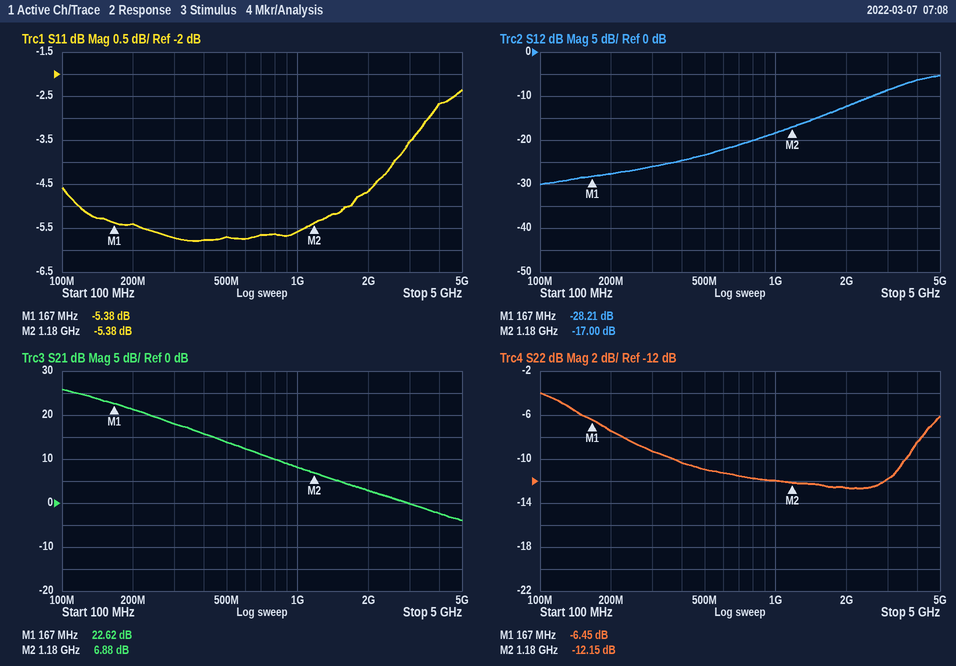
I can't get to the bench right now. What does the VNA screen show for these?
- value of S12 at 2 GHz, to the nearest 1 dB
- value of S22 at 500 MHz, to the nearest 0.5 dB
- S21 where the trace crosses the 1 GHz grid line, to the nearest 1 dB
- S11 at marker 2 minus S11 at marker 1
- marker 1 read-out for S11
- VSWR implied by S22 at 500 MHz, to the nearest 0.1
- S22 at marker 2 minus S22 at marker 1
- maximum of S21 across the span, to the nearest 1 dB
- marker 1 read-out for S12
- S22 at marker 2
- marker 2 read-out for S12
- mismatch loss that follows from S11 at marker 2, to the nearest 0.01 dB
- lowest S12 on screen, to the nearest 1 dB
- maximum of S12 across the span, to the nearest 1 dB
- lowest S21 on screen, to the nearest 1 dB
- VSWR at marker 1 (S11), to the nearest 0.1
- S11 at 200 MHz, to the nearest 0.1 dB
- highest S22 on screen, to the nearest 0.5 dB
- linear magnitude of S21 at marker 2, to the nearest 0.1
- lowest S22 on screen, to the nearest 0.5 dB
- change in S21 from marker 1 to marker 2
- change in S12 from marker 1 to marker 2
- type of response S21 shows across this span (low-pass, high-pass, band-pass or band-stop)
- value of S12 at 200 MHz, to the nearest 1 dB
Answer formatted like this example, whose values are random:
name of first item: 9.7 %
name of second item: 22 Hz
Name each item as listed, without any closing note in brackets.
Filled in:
value of S12 at 2 GHz, to the nearest 1 dB: -12 dB
value of S22 at 500 MHz, to the nearest 0.5 dB: -11.0 dB
S21 where the trace crosses the 1 GHz grid line, to the nearest 1 dB: 8 dB
S11 at marker 2 minus S11 at marker 1: 0.00 dB
marker 1 read-out for S11: -5.38 dB
VSWR implied by S22 at 500 MHz, to the nearest 0.1: 1.8
S22 at marker 2 minus S22 at marker 1: -5.70 dB
maximum of S21 across the span, to the nearest 1 dB: 26 dB
marker 1 read-out for S12: -28.21 dB
S22 at marker 2: -12.15 dB
marker 2 read-out for S12: -17.00 dB
mismatch loss that follows from S11 at marker 2, to the nearest 0.01 dB: 1.49 dB
lowest S12 on screen, to the nearest 1 dB: -30 dB
maximum of S12 across the span, to the nearest 1 dB: -5 dB
lowest S21 on screen, to the nearest 1 dB: -4 dB
VSWR at marker 1 (S11), to the nearest 0.1: 3.3
S11 at 200 MHz, to the nearest 0.1 dB: -5.4 dB
highest S22 on screen, to the nearest 0.5 dB: -4.0 dB
linear magnitude of S21 at marker 2, to the nearest 0.1: 2.2
lowest S22 on screen, to the nearest 0.5 dB: -12.5 dB
change in S21 from marker 1 to marker 2: -15.74 dB
change in S12 from marker 1 to marker 2: 11.21 dB
type of response S21 shows across this span: low-pass
value of S12 at 200 MHz, to the nearest 1 dB: -28 dB
